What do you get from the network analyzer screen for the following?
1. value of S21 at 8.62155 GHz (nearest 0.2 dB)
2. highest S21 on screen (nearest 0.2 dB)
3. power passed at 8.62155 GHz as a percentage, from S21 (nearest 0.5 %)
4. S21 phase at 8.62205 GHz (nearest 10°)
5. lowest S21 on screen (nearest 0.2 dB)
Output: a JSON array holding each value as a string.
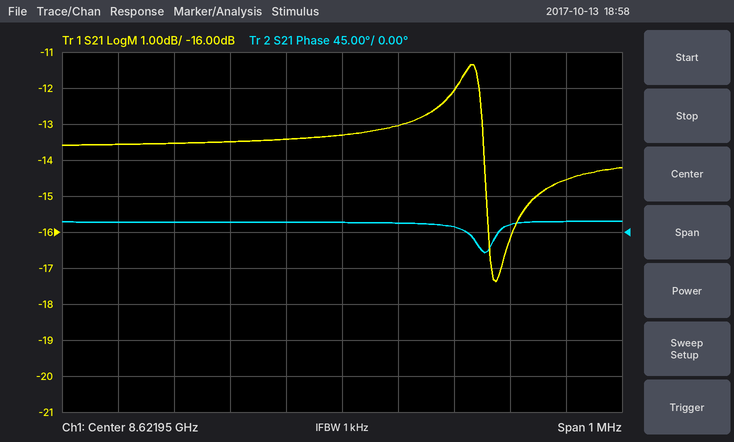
["-13.6 dB", "-11.4 dB", "4.5 %", "10°", "-17.4 dB"]
